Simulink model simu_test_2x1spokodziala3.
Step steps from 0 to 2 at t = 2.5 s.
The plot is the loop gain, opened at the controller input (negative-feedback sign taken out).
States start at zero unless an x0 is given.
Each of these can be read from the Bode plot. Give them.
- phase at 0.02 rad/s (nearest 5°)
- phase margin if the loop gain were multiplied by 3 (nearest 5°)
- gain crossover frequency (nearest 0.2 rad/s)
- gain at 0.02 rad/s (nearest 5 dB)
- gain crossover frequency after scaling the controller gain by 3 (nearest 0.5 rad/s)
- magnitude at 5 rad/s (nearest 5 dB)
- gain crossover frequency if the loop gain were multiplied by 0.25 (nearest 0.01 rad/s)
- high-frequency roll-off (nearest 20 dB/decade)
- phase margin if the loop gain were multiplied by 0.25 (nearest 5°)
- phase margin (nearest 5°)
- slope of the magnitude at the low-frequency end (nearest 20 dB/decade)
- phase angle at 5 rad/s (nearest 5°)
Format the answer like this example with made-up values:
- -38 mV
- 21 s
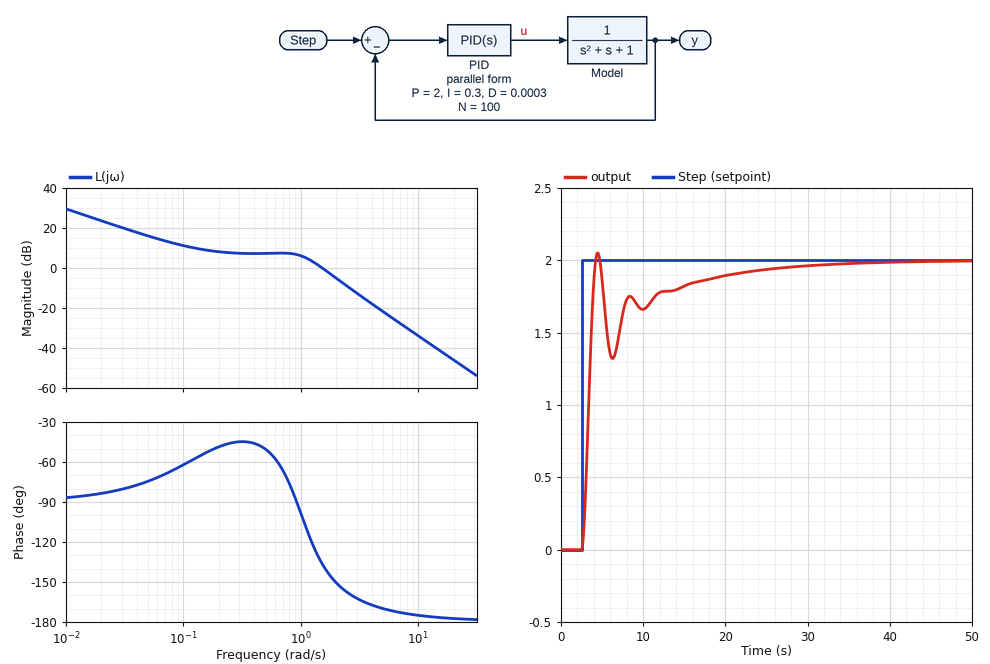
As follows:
- -85°
- 20°
- 1.6 rad/s
- 25 dB
- 2.5 rad/s
- -20 dB
- 0.09 rad/s
- -40 dB/decade
- 115°
- 45°
- -20 dB/decade
- -170°
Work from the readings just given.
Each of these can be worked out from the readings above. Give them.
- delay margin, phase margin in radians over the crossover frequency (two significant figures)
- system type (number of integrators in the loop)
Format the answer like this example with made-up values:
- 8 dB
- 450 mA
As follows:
- 0.49 s
- 1
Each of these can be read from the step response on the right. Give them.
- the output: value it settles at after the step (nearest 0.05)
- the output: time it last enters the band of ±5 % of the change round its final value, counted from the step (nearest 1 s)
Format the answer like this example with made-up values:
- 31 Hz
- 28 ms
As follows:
- 2.00
- 18 s
